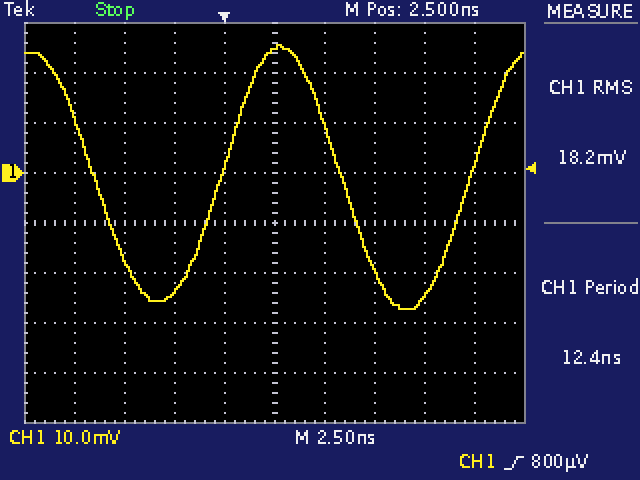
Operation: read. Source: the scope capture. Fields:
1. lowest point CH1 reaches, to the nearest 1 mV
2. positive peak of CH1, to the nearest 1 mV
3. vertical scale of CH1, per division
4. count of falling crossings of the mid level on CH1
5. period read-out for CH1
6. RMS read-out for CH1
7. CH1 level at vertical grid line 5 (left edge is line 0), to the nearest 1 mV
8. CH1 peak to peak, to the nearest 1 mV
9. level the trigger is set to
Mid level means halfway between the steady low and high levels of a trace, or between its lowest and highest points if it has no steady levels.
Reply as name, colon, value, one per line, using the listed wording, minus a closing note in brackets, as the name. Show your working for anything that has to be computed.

lowest point CH1 reaches, to the nearest 1 mV: -27 mV
positive peak of CH1, to the nearest 1 mV: 26 mV
vertical scale of CH1, per division: 10 mV
count of falling crossings of the mid level on CH1: 2
period read-out for CH1: 12.4 ns
RMS read-out for CH1: 18.2 mV
CH1 level at vertical grid line 5 (left edge is line 0), to the nearest 1 mV: 25 mV
CH1 peak to peak, to the nearest 1 mV: 26 mV − (-27 mV) = 53 mV
level the trigger is set to: 800 µV
